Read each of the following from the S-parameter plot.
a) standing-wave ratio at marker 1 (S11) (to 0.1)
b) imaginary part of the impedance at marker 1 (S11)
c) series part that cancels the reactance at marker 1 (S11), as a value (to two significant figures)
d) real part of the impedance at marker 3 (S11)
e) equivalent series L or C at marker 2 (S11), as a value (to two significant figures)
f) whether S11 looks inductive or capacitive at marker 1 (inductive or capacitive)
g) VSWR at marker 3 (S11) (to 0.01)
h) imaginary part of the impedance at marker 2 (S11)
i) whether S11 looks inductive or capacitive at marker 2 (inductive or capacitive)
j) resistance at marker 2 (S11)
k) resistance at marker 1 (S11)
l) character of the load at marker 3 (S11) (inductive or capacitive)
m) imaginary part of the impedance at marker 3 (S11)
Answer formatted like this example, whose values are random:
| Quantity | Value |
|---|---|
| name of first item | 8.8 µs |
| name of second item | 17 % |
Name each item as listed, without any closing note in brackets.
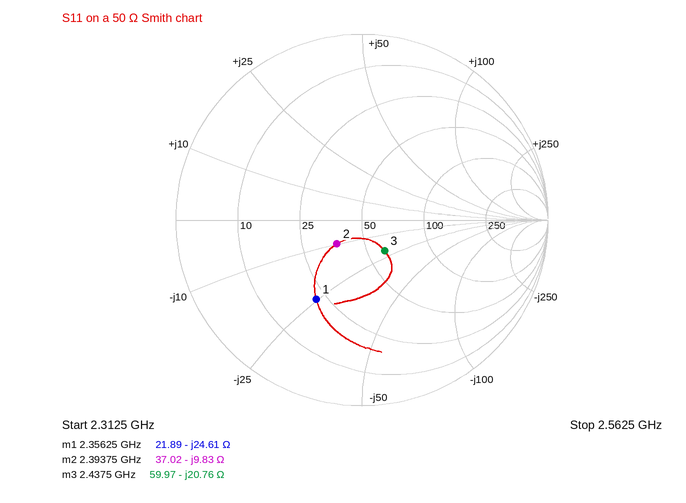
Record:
| Quantity | Value |
|---|---|
| standing-wave ratio at marker 1 (S11) | 2.9 |
| imaginary part of the impedance at marker 1 | -24.61 Ω |
| series part that cancels the reactance at marker 1 (S11), as a value | 1.7 nH |
| real part of the impedance at marker 3 | 59.97 Ω |
| equivalent series L or C at marker 2 (S11), as a value | 6.8 pF |
| whether S11 looks inductive or capacitive at marker 1 | capacitive |
| VSWR at marker 3 (S11) | 1.52 |
| imaginary part of the impedance at marker 2 | -9.83 Ω |
| whether S11 looks inductive or capacitive at marker 2 | capacitive |
| resistance at marker 2 | 37.02 Ω |
| resistance at marker 1 | 21.89 Ω |
| character of the load at marker 3 (S11) | capacitive |
| imaginary part of the impedance at marker 3 | -20.76 Ω |
